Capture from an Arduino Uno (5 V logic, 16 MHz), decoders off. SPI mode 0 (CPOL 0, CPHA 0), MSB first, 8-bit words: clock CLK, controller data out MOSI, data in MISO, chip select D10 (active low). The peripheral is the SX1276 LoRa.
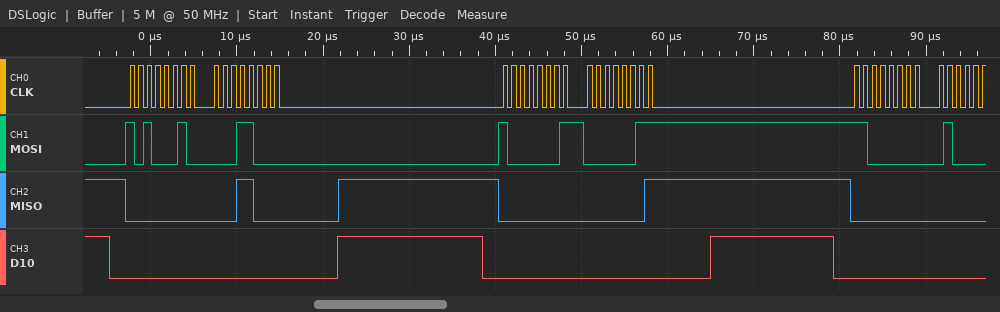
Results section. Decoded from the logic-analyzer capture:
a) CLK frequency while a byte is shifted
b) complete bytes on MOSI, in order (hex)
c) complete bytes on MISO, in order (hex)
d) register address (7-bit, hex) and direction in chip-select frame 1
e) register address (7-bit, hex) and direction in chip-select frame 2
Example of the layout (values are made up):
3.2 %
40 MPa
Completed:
1 MHz
A2 18 81 03 C0
00 18 00 01 00
0x22 write
0x01 write
